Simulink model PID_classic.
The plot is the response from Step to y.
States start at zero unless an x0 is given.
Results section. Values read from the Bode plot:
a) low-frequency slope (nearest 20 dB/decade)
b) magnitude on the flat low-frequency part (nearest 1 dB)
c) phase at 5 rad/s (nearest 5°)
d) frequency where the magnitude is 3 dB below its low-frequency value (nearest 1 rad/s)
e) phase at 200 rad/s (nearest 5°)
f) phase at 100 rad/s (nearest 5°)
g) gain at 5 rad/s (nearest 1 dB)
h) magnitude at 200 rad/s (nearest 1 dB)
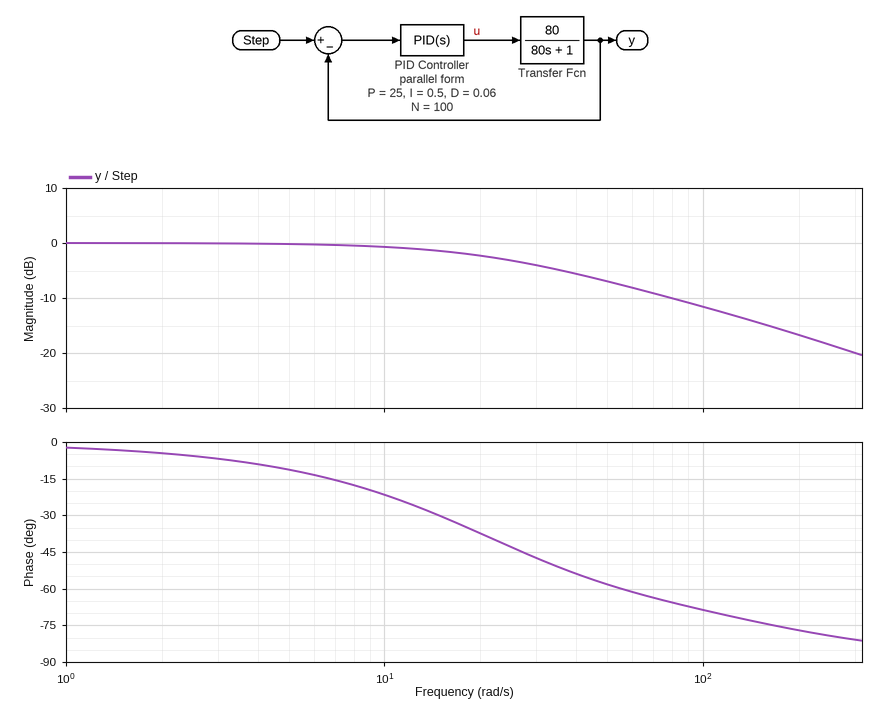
0 dB/decade
0 dB
-10°
24 rad/s
-75°
-70°
0 dB
-17 dB
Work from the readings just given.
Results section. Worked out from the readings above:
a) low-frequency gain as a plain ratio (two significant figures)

1.0
